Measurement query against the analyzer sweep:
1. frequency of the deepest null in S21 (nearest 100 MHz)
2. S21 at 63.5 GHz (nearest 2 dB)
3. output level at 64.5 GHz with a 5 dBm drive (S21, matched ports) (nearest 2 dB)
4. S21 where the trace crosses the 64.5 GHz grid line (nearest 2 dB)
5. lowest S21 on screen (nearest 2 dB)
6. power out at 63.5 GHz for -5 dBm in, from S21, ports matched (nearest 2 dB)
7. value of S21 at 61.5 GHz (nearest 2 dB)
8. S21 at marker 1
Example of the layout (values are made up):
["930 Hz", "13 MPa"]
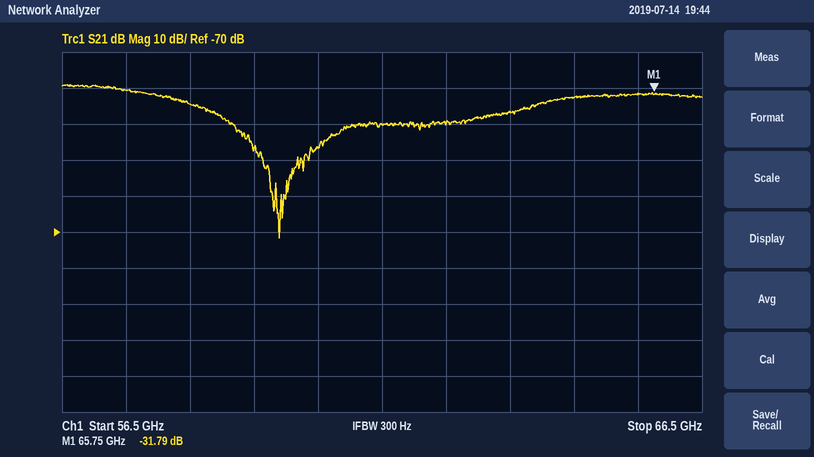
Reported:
["59.9 GHz", "-36 dB", "-28 dBm", "-32 dB", "-72 dB", "-42 dBm", "-40 dB", "-31.79 dB"]
